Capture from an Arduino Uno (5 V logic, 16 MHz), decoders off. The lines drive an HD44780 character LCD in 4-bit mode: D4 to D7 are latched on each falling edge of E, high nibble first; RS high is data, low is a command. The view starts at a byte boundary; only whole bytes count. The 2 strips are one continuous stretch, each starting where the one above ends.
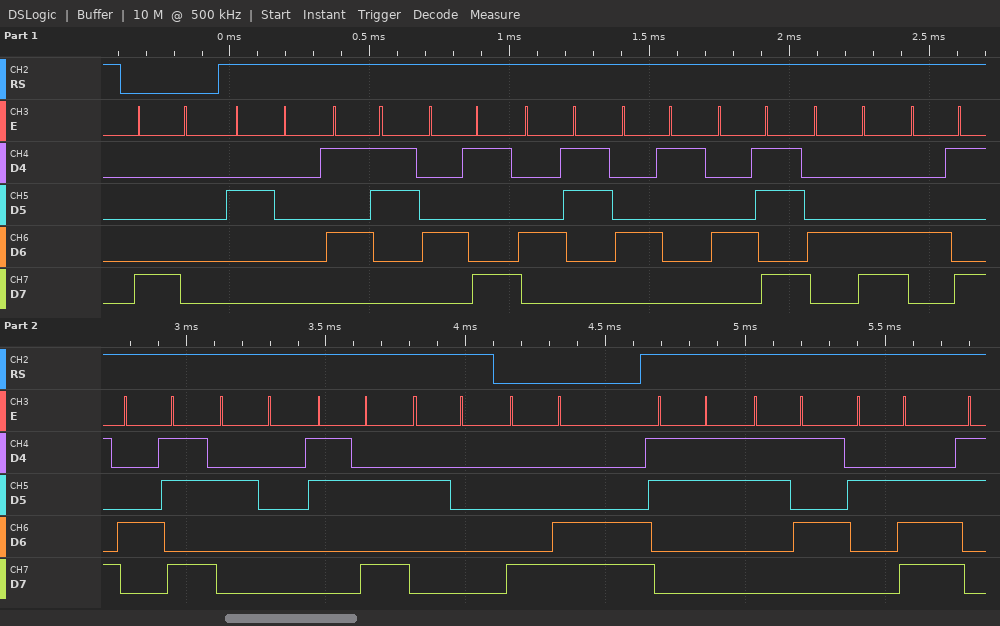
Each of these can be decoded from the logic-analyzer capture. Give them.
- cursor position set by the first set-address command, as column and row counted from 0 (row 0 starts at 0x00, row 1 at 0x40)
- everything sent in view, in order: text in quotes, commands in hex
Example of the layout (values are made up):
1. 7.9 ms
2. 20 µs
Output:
1. column 0, row 0
2. 0x80 " SICAKLIK : " 0x8C "35."
